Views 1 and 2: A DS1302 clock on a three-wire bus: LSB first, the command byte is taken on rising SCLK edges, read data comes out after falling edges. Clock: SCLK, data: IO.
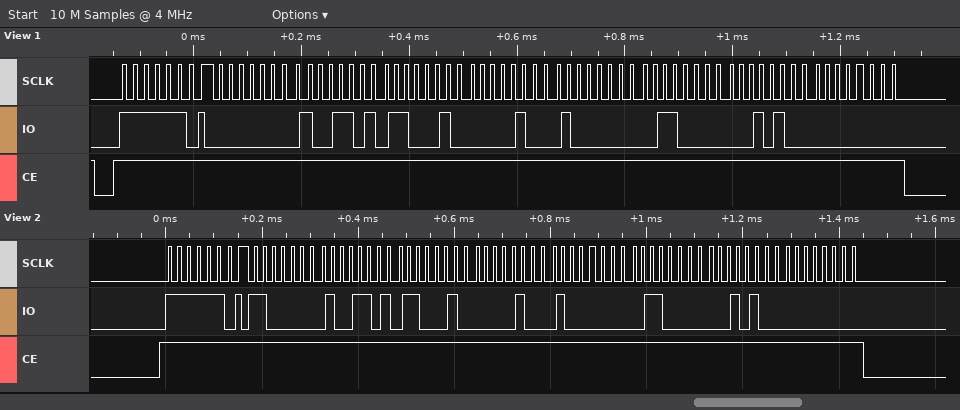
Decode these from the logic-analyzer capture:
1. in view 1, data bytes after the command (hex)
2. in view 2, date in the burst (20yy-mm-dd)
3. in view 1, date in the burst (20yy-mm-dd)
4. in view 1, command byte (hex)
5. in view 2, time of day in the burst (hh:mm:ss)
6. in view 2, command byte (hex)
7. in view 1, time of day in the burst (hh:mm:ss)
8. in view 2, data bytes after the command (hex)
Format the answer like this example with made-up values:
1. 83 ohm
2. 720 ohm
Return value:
1. 00 59 23 10 01 06 14 00
2. 2014-01-10
3. 2014-01-10
4. 0xBF
5. 23:59:03
6. 0xBF
7. 23:59:00
8. 03 59 23 10 01 06 14 00
